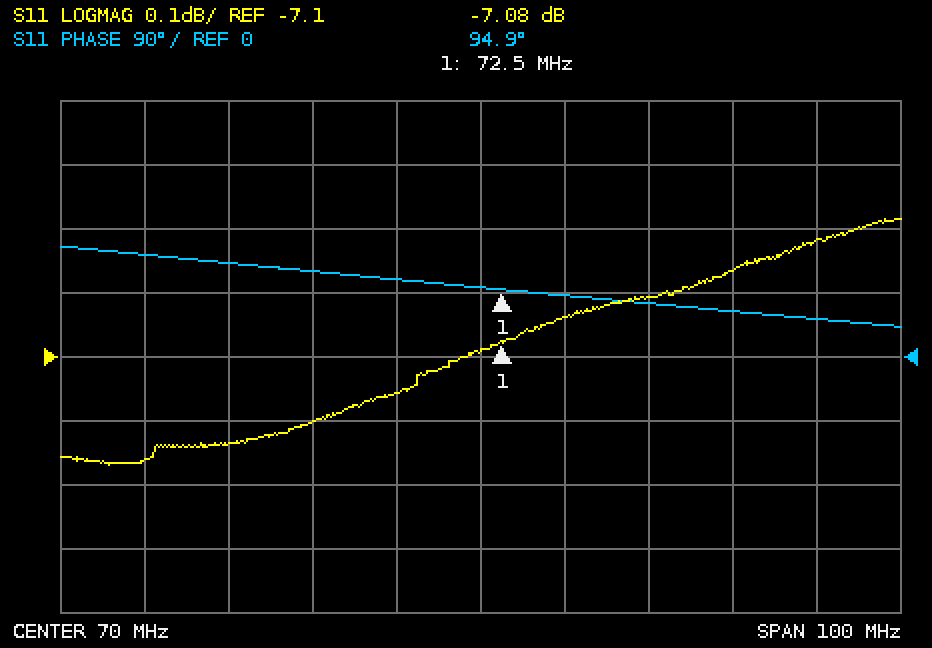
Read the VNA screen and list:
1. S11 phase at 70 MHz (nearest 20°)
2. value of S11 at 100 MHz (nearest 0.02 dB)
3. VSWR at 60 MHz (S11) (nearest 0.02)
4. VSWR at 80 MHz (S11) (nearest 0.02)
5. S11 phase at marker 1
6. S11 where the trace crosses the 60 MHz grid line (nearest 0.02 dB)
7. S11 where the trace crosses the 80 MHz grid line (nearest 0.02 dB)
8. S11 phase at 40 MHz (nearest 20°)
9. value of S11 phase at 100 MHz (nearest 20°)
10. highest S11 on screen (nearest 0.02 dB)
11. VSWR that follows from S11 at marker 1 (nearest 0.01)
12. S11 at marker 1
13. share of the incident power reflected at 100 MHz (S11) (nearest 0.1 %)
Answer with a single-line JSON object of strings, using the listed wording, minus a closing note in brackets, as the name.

{"S11 phase at 70 MHz": "100°", "value of S11 at 100 MHz": "-6.96 dB", "VSWR at 60 MHz (S11)": "2.56", "VSWR at 80 MHz (S11)": "2.60", "S11 phase at marker 1": "94.9°", "S11 where the trace crosses the 60 MHz grid line": "-7.16 dB", "S11 where the trace crosses the 80 MHz grid line": "-7.04 dB", "S11 phase at 40 MHz": "140°", "value of S11 phase at 100 MHz": "60°", "highest S11 on screen": "-6.88 dB", "VSWR that follows from S11 at marker 1": "2.59", "S11 at marker 1": "-7.08 dB", "share of the incident power reflected at 100 MHz (S11)": "20.1 %"}
